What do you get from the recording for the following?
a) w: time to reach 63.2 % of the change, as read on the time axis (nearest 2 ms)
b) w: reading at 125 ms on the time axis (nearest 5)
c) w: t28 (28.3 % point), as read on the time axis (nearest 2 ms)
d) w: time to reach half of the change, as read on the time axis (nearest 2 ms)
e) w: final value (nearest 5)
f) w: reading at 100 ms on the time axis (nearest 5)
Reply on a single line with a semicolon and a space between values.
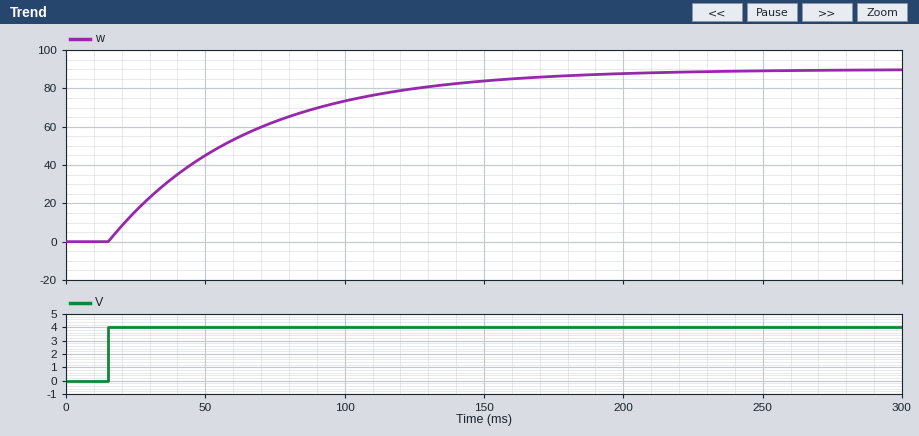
66 ms; 80; 32 ms; 50 ms; 90; 75
